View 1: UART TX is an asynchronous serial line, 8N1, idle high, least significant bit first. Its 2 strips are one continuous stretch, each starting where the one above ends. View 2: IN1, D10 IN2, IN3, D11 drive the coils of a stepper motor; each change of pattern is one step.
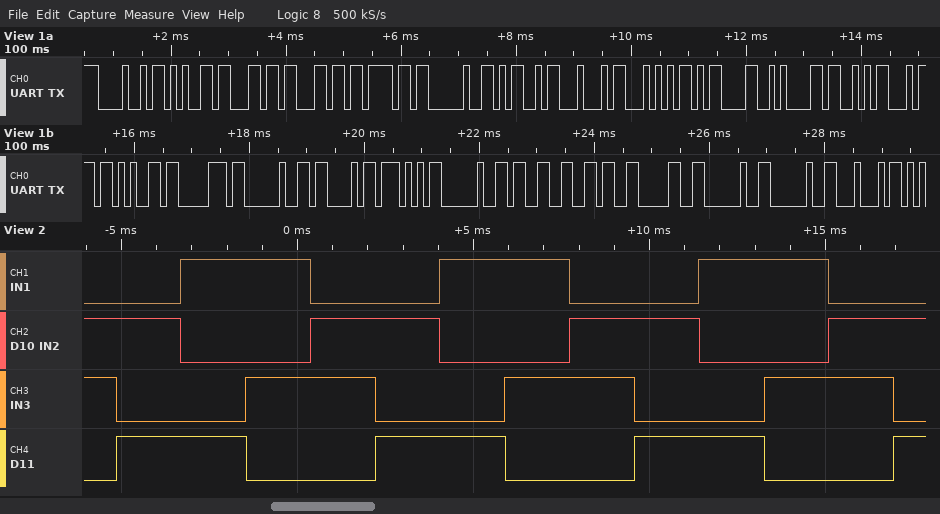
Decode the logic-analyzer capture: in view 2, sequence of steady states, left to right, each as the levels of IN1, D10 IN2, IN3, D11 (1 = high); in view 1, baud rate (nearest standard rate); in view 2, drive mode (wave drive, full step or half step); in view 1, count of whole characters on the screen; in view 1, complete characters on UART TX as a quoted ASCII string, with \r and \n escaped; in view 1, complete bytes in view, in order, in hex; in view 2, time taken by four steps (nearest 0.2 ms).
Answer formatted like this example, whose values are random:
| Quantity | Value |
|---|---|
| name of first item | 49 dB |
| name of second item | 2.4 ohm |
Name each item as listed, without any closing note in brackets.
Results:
| Quantity | Value |
|---|---|
| in view 2, sequence of steady states, left to right, each as the levels of IN1, D10 IN2, IN3, D11 | 0110 0101 1001 1010 0110 0101 1001 1010 0110 0101 1001 1010 0110 0101 |
| in view 1, baud rate | 9600 baud |
| in view 2, drive mode | full step |
| in view 1, count of whole characters on the screen | 25 |
| in view 1, complete characters on UART TX as a quoted ASCII string, with \r and \n escaped | "Hello MDT\r\nStep CW 360  D" |
| in view 1, complete bytes in view, in order, in hex | 48 65 6C 6C 6F 20 4D 44 54 0D 0A 53 74 65 70 20 43 57 20 33 36 30 20 20 44 |
| in view 2, time taken by four steps | 7.4 ms |
